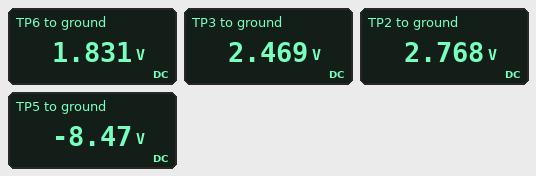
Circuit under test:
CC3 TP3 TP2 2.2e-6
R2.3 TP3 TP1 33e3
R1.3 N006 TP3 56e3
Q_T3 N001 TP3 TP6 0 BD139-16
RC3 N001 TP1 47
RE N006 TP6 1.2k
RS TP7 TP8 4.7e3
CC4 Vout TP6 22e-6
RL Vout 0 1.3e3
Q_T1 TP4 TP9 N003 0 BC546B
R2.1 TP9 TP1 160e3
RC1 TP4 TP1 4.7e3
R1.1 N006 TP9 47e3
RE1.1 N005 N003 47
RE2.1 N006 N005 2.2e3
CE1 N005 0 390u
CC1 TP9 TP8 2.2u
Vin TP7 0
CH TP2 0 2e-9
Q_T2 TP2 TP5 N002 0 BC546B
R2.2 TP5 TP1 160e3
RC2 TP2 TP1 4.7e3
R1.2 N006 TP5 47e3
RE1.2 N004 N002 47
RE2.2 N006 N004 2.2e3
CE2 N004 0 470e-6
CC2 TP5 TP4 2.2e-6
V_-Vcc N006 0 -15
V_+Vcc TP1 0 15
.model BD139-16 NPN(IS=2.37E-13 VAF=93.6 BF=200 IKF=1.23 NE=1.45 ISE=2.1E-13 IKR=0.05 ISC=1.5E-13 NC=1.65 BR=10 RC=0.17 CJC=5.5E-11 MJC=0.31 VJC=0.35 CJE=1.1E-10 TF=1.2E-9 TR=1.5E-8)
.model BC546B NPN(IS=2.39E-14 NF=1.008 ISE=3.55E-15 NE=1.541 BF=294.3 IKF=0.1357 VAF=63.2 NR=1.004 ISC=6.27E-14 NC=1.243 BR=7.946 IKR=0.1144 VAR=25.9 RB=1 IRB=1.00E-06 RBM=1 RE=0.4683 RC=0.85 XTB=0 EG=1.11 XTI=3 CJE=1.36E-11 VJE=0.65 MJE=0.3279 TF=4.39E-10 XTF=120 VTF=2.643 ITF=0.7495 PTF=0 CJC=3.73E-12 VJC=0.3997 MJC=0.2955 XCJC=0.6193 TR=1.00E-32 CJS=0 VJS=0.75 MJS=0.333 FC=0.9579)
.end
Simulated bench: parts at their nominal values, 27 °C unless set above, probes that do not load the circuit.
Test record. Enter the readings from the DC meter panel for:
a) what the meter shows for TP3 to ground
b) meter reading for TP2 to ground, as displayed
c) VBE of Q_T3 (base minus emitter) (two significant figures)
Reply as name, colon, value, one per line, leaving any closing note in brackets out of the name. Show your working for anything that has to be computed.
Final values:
what the meter shows for TP3 to ground: 2.469 V
meter reading for TP2 to ground, as displayed: 2.768 V
VBE of Q_T3 (base minus emitter): 2.469 V - 1.831 V = 640 mV
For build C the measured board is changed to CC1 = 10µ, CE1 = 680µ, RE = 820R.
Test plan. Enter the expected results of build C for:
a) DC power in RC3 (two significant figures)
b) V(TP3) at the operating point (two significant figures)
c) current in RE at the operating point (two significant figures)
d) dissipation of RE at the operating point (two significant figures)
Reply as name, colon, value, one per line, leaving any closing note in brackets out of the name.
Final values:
DC power in RC3: 18 mW
V(TP3) at the operating point: 1.9 V
current in RE at the operating point: 20 mA
dissipation of RE at the operating point: 320 mW
